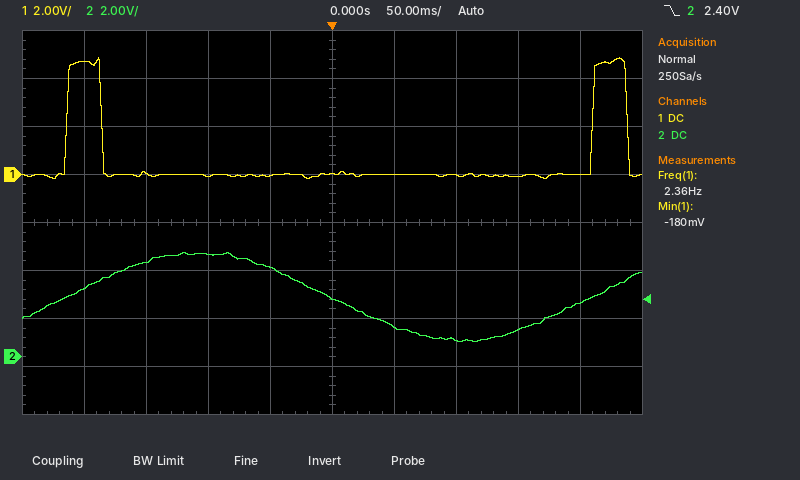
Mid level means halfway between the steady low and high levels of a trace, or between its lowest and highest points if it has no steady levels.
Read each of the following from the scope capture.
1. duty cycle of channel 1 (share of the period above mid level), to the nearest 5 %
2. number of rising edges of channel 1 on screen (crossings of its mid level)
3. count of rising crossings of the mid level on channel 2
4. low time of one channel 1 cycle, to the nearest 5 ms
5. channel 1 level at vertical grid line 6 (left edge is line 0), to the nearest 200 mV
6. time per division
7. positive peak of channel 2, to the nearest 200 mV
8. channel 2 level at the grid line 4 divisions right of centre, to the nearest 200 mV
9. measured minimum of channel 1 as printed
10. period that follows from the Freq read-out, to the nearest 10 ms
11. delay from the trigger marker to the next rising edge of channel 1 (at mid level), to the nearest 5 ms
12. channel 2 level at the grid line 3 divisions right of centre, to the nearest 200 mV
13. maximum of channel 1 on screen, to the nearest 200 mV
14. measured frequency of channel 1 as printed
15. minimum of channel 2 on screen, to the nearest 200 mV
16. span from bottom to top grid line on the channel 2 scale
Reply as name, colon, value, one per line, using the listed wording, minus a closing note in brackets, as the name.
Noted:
duty cycle of channel 1 (share of the period above mid level), to the nearest 5 %: 5 %
number of rising edges of channel 1 on screen: 2
count of rising crossings of the mid level on channel 2: 2
low time of one channel 1 cycle, to the nearest 5 ms: 395 ms
channel 1 level at vertical grid line 6 (left edge is line 0), to the nearest 200 mV: 0.0 V
time per division: 50 ms
positive peak of channel 2, to the nearest 200 mV: 4.4 V
channel 2 level at the grid line 4 divisions right of centre, to the nearest 200 mV: 2.2 V
measured minimum of channel 1 as printed: -180 mV
period that follows from the Freq read-out, to the nearest 10 ms: 420 ms
delay from the trigger marker to the next rising edge of channel 1 (at mid level), to the nearest 5 ms: 210 ms
channel 2 level at the grid line 3 divisions right of centre, to the nearest 200 mV: 1.2 V
maximum of channel 1 on screen, to the nearest 200 mV: 4.8 V
measured frequency of channel 1 as printed: 2.36 Hz
minimum of channel 2 on screen, to the nearest 200 mV: 600 mV
span from bottom to top grid line on the channel 2 scale: 16 V
